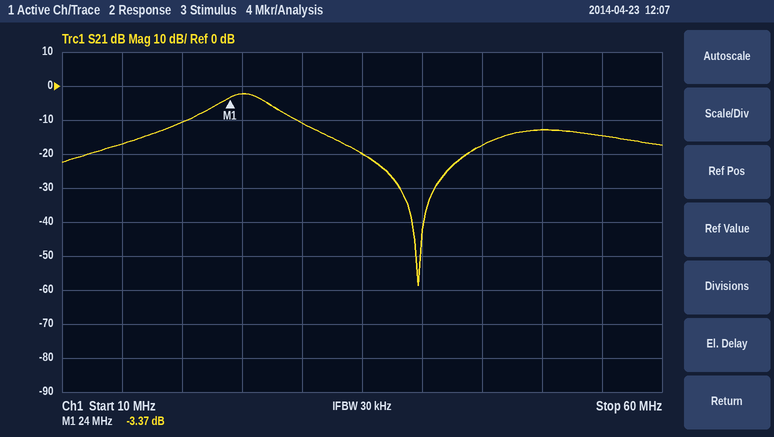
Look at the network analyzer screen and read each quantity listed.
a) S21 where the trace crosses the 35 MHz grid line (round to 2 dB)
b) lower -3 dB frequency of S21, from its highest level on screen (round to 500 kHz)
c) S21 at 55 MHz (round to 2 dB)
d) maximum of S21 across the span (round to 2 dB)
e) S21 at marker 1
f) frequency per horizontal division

-20 dB
23.0 MHz
-14 dB
-2 dB
-3.37 dB
5 MHz
